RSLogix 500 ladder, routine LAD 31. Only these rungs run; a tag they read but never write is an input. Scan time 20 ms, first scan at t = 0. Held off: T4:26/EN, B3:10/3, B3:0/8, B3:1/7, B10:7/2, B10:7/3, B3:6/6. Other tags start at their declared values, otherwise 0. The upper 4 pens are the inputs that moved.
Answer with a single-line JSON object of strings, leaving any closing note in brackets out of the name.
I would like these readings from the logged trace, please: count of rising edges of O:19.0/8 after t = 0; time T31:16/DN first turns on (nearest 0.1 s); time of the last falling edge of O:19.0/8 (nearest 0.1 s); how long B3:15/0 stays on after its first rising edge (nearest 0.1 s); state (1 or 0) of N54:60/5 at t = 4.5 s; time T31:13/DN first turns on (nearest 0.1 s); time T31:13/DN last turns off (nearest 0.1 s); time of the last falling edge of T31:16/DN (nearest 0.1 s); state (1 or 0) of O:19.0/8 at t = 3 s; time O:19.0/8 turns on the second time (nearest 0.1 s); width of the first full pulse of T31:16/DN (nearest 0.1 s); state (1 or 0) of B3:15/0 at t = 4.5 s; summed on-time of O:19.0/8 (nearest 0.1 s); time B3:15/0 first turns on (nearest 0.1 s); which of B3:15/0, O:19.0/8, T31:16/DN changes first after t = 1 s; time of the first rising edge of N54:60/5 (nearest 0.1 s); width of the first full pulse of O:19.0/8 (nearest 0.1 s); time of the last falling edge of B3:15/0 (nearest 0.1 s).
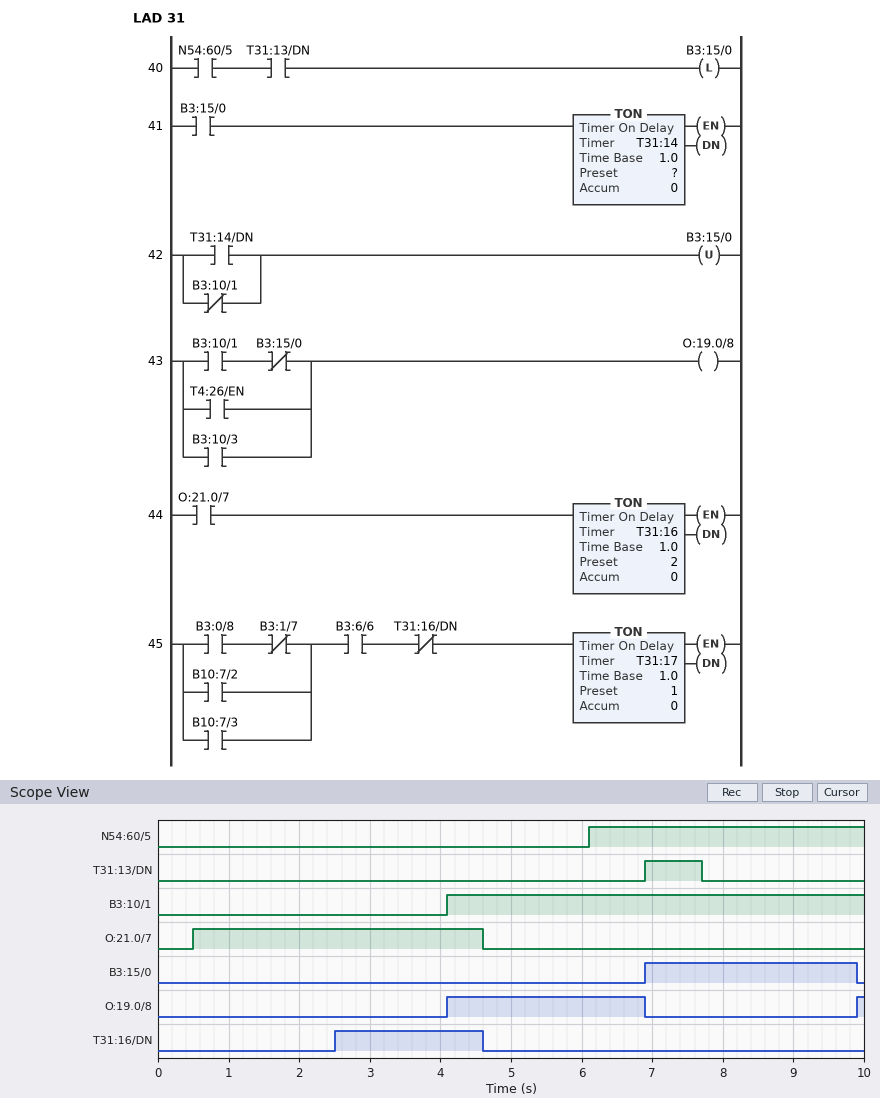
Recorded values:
{"count of rising edges of O:19.0/8 after t = 0": "2", "time T31:16/DN first turns on": "2.5 s", "time of the last falling edge of O:19.0/8": "6.9 s", "how long B3:15/0 stays on after its first rising edge": "3.0 s", "state (1 or 0) of N54:60/5 at t = 4.5 s": "0", "time T31:13/DN first turns on": "6.9 s", "time T31:13/DN last turns off": "7.7 s", "time of the last falling edge of T31:16/DN": "4.6 s", "state (1 or 0) of O:19.0/8 at t = 3 s": "0", "time O:19.0/8 turns on the second time": "9.9 s", "width of the first full pulse of T31:16/DN": "2.1 s", "state (1 or 0) of B3:15/0 at t = 4.5 s": "0", "summed on-time of O:19.0/8": "2.9 s", "time B3:15/0 first turns on": "6.9 s", "which of B3:15/0, O:19.0/8, T31:16/DN changes first after t = 1 s": "T31:16/DN", "time of the first rising edge of N54:60/5": "6.1 s", "width of the first full pulse of O:19.0/8": "2.8 s", "time of the last falling edge of B3:15/0": "9.9 s"}
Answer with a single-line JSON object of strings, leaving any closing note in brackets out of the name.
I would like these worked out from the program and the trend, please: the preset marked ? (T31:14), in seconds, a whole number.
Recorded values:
{"the preset marked ? (T31:14), in seconds, a whole number": "3 s"}
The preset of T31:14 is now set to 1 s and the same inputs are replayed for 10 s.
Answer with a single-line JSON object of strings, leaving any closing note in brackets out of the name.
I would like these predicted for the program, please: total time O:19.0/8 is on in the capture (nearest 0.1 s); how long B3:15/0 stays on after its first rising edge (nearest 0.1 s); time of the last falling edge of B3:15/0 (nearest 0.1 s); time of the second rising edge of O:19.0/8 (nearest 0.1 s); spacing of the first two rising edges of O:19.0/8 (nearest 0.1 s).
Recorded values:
{"total time O:19.0/8 is on in the capture": "4.9 s", "how long B3:15/0 stays on after its first rising edge": "1.0 s", "time of the last falling edge of B3:15/0": "7.9 s", "time of the second rising edge of O:19.0/8": "7.9 s", "spacing of the first two rising edges of O:19.0/8": "3.8 s"}
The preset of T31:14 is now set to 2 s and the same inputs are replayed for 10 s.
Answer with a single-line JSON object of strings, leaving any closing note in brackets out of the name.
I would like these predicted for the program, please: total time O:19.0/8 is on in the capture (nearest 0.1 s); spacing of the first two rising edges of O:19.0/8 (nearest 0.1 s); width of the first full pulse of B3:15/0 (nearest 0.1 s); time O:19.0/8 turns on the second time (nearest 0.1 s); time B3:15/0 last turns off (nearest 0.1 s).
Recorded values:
{"total time O:19.0/8 is on in the capture": "3.9 s", "spacing of the first two rising edges of O:19.0/8": "4.8 s", "width of the first full pulse of B3:15/0": "2.0 s", "time O:19.0/8 turns on the second time": "8.9 s", "time B3:15/0 last turns off": "8.9 s"}
